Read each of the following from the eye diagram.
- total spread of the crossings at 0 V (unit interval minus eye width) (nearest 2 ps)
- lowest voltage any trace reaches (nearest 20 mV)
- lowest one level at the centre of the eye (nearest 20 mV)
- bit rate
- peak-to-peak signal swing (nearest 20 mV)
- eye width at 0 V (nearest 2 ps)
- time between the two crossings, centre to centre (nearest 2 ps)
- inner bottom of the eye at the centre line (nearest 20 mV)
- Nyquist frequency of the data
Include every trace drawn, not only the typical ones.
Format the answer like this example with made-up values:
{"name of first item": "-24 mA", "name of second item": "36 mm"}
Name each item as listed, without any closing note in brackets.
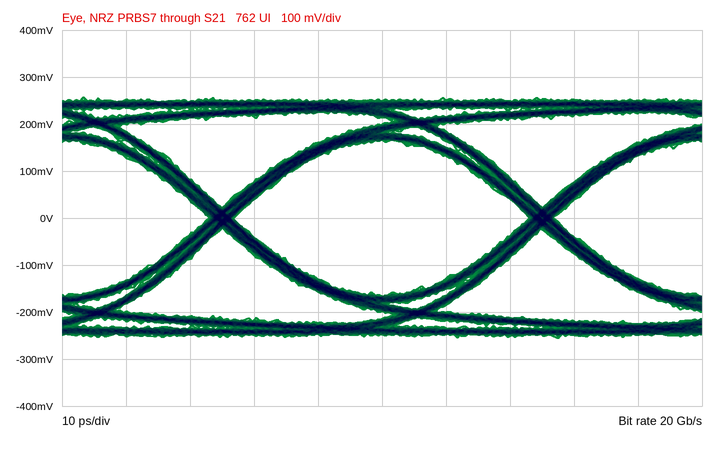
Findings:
{"total spread of the crossings at 0 V (unit interval minus eye width)": "4 ps", "lowest voltage any trace reaches": "-260 mV", "lowest one level at the centre of the eye": "160 mV", "bit rate": "20 Gb/s", "peak-to-peak signal swing": "520 mV", "eye width at 0 V": "46 ps", "time between the two crossings, centre to centre": "50 ps", "inner bottom of the eye at the centre line": "-160 mV", "Nyquist frequency of the data": "10 GHz"}
